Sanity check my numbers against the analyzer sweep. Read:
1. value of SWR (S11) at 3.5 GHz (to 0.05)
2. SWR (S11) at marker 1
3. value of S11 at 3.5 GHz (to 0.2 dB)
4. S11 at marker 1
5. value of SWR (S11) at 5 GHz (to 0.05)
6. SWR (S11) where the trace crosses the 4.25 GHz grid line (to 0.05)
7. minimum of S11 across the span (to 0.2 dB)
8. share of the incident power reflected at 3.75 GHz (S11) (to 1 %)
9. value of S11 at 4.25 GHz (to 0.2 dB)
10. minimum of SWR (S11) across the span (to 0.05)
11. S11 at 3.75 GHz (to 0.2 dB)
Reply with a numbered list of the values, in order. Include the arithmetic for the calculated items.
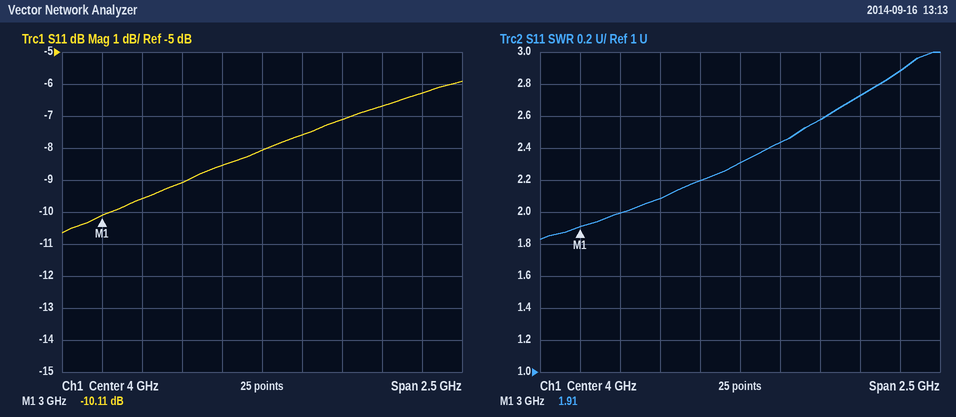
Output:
1. 2.10
2. 1.91
3. -9.0 dB
4. -10.11 dB
5. 2.90
6. 2.45
7. -10.6 dB
8. 10^(-8.6/10) ≈ 14 %
9. -7.6 dB
10. 1.85
11. -8.6 dB
